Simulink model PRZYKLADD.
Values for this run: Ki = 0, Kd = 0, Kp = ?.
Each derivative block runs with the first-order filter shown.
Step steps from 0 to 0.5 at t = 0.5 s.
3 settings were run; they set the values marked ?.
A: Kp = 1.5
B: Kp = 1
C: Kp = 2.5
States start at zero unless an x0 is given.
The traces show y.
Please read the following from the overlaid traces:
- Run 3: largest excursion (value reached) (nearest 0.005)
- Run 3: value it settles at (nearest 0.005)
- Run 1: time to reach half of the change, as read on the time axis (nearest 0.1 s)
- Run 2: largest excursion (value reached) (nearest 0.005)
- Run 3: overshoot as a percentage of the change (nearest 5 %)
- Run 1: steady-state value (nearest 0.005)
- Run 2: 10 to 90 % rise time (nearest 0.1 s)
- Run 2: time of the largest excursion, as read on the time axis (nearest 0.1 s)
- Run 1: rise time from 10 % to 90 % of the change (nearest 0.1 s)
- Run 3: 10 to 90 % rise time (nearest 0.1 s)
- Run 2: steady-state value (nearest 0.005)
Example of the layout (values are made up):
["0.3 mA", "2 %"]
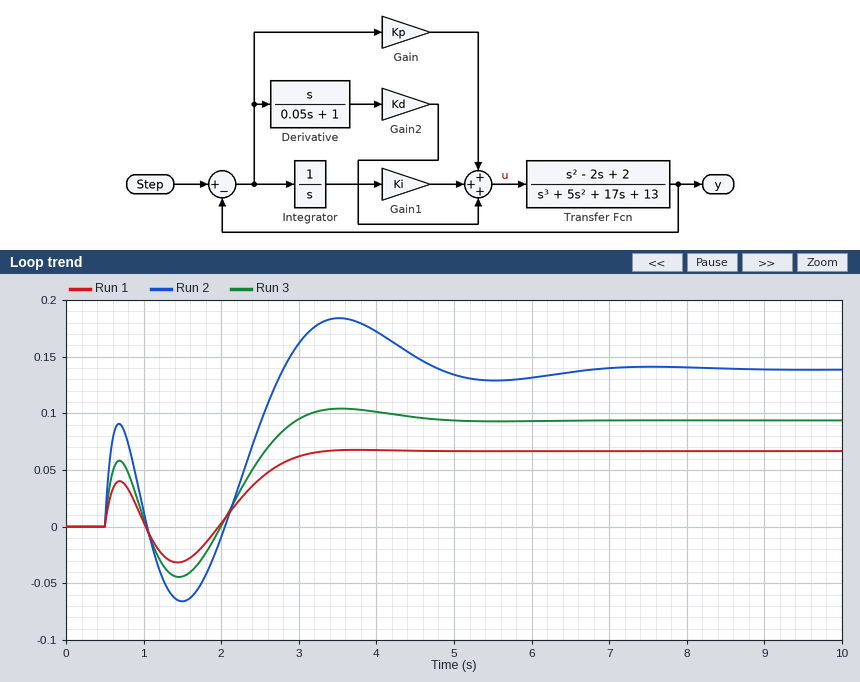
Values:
["0.105", "0.095", "0.6 s", "0.185", "10 %", "0.065", "2.2 s", "3.5 s", "2.4 s", "2.3 s", "0.140"]
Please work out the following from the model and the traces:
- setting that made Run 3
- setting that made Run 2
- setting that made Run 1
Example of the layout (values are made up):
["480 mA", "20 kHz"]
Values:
["A", "C", "B"]
